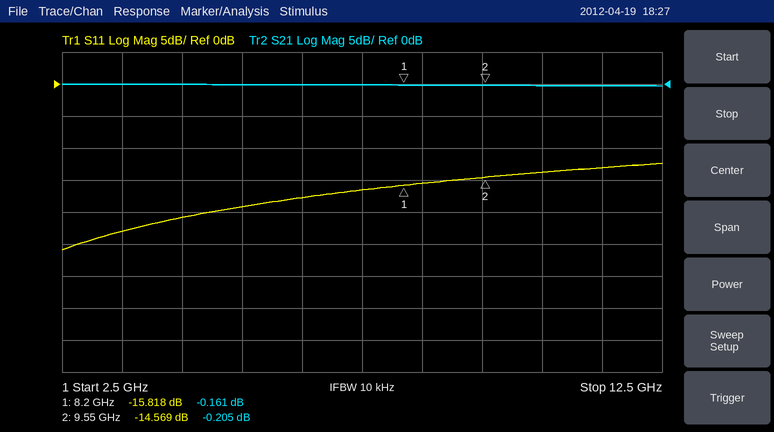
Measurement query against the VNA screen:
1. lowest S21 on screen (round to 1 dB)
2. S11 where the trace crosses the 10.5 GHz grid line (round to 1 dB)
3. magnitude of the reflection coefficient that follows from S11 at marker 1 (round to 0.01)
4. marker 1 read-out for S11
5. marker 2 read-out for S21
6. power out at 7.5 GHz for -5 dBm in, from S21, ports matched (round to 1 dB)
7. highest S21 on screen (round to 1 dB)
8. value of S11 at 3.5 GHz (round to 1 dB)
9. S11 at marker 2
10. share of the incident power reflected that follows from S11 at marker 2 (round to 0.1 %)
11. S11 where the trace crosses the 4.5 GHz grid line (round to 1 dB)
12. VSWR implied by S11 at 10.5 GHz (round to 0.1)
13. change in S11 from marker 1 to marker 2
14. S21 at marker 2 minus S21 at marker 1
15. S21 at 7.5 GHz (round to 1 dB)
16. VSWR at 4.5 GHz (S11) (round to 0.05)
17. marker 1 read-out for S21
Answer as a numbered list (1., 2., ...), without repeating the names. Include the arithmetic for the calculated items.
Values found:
1. 0 dB
2. -14 dB
3. 10^(-15.818/20) ≈ 0.16
4. -15.818 dB
5. -0.205 dB
6. -5 dBm + (0 dB) = -5 dBm
7. 0 dB
8. -23 dB
9. -14.569 dB
10. 10^(-14.569/10) ≈ 3.5 %
11. -21 dB
12. |Γ| = 10^(-14/20) = 0.1995; VSWR = (1 + 0.1995)/(1 − 0.1995) ≈ 1.5
13. -14.569 − (-15.818) = 1.249 dB
14. -0.205 − (-0.161) = -0.044 dB
15. 0 dB
16. |Γ| = 10^(-21/20) = 0.0891; VSWR = (1 + 0.0891)/(1 − 0.0891) ≈ 1.20
17. -0.161 dB
